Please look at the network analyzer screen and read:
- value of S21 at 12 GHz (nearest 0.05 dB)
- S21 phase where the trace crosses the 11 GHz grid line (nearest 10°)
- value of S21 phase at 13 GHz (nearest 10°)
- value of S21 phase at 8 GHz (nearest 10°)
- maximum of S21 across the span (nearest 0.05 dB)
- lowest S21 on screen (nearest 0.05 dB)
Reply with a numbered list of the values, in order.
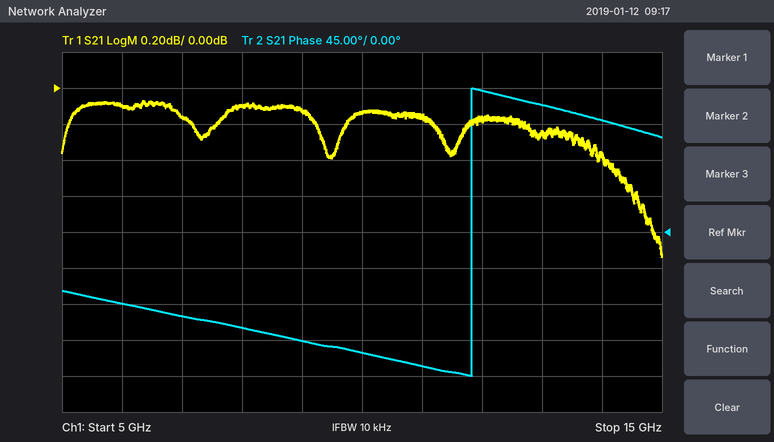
1. -0.15 dB
2. -170°
3. 160°
4. -120°
5. -0.05 dB
6. -0.95 dB
